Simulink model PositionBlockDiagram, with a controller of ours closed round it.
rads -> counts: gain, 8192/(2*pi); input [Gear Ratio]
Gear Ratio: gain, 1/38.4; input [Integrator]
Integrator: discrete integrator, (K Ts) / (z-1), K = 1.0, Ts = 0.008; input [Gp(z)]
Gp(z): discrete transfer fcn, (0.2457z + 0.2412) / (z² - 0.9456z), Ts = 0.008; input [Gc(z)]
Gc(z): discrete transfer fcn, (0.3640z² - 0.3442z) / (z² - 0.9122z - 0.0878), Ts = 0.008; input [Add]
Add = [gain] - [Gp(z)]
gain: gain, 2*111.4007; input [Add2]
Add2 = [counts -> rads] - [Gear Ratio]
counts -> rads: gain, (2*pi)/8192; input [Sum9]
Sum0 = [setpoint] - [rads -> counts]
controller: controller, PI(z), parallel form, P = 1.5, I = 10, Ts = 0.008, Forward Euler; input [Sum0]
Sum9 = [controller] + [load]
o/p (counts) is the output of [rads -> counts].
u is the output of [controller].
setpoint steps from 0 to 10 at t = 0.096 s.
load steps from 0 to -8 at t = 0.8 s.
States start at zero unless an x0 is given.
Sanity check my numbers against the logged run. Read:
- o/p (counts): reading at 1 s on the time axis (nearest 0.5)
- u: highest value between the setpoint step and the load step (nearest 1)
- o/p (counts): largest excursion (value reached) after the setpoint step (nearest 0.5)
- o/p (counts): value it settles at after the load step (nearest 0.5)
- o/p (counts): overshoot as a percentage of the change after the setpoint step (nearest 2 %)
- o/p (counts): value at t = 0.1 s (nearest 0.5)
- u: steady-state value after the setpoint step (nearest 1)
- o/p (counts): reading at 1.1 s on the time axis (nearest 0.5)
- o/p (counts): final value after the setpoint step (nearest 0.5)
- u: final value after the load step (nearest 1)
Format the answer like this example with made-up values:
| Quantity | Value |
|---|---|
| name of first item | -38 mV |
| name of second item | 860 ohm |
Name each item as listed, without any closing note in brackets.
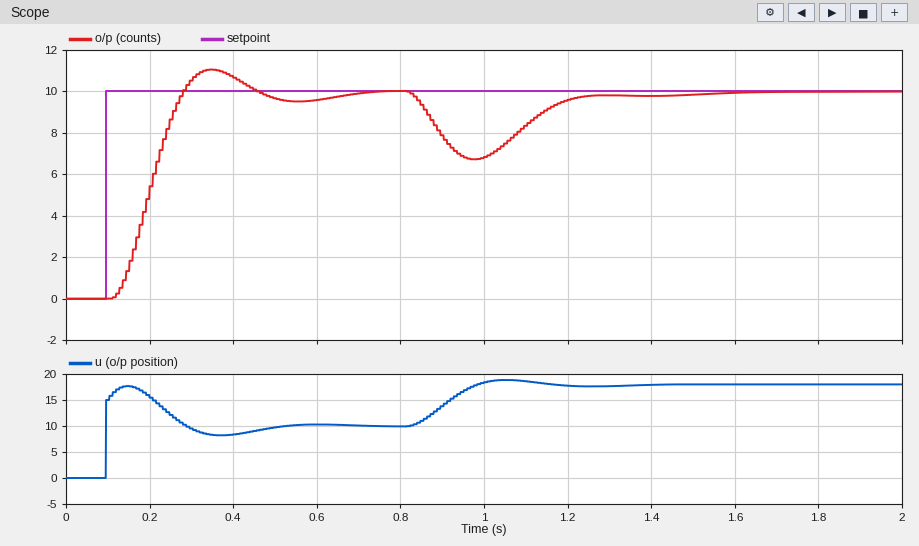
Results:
| Quantity | Value |
|---|---|
| o/p (counts): reading at 1 s on the time axis | 7.0 |
| u: highest value between the setpoint step and the load step | 18 |
| o/p (counts): largest excursion (value reached) after the setpoint step | 11.0 |
| o/p (counts): value it settles at after the load step | 10.0 |
| o/p (counts): overshoot as a percentage of the change after the setpoint step | 10 % |
| o/p (counts): value at t = 0.1 s | 0.0 |
| u: steady-state value after the setpoint step | 10 |
| o/p (counts): reading at 1.1 s on the time axis | 8.5 |
| o/p (counts): final value after the setpoint step | 10.0 |
| u: final value after the load step | 18 |
